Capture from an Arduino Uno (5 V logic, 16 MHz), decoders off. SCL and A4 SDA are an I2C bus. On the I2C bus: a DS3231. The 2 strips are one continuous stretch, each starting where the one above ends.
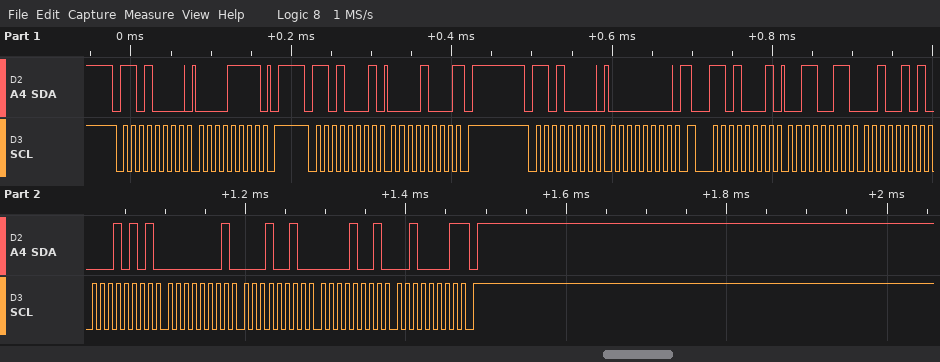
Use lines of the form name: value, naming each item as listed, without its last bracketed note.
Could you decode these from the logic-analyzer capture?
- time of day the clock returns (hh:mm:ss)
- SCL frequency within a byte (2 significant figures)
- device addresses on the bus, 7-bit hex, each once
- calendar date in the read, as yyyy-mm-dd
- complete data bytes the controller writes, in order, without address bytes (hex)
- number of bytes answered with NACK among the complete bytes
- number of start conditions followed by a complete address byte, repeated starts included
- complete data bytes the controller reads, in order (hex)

time of day the clock returns: 15:25:33
SCL frequency within a byte: 100 kHz
device addresses on the bus, 7-bit hex, each once: 0x68
calendar date in the read, as yyyy-mm-dd: 2021-09-12
complete data bytes the controller writes, in order, without address bytes: 0F 00
number of bytes answered with NACK among the complete bytes: 2
number of start conditions followed by a complete address byte, repeated starts included: 4
complete data bytes the controller reads, in order: 08 33 25 15 01 12 09 21
